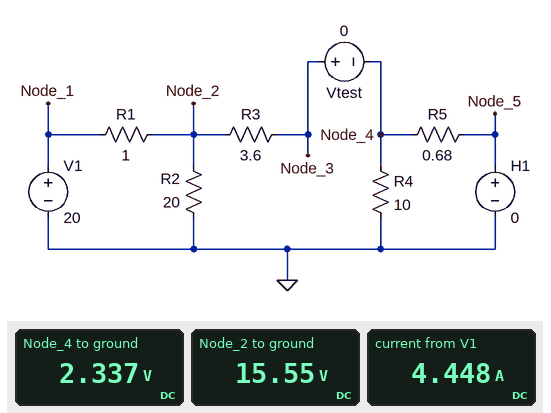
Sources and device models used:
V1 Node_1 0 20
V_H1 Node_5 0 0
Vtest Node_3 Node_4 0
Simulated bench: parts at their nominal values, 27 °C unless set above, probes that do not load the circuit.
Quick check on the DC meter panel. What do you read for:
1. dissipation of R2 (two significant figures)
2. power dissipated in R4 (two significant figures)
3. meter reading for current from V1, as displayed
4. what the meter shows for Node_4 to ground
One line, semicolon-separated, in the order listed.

12 W; 550 mW; 4.448 A; 2.337 V
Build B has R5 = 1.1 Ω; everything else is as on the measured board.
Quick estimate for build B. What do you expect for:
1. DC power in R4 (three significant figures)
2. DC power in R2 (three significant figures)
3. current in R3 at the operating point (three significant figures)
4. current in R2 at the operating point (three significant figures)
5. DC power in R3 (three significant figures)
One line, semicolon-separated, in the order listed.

1.16 W; 12.4 W; 3.44 A; 789 mA; 42.5 W
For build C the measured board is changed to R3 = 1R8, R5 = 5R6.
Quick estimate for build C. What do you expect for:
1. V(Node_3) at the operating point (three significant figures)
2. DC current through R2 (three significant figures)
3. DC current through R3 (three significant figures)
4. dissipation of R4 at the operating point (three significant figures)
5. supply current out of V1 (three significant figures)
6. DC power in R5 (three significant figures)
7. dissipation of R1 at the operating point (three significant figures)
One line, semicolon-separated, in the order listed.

10.8 V; 809 mA; 3.00 A; 11.6 W; 3.81 A; 20.8 W; 14.5 W
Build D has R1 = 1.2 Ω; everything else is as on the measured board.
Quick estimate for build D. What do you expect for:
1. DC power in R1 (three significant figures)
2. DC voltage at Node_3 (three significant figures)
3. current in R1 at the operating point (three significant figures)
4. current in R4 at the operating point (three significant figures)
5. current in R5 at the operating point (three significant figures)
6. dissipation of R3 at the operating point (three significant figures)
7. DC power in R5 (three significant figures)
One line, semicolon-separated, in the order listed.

21.8 W; 2.24 V; 4.26 A; 224 mA; 3.29 A; 44.5 W; 7.36 W
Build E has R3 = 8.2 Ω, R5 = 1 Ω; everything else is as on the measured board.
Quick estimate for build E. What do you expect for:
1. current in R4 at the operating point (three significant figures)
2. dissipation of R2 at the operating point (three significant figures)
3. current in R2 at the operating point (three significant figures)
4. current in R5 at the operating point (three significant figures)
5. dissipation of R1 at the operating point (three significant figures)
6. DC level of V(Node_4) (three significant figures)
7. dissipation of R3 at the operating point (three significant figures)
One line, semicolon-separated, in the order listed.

172 mA; 14.9 W; 862 mA; 1.72 A; 7.59 W; 1.72 V; 29.4 W
